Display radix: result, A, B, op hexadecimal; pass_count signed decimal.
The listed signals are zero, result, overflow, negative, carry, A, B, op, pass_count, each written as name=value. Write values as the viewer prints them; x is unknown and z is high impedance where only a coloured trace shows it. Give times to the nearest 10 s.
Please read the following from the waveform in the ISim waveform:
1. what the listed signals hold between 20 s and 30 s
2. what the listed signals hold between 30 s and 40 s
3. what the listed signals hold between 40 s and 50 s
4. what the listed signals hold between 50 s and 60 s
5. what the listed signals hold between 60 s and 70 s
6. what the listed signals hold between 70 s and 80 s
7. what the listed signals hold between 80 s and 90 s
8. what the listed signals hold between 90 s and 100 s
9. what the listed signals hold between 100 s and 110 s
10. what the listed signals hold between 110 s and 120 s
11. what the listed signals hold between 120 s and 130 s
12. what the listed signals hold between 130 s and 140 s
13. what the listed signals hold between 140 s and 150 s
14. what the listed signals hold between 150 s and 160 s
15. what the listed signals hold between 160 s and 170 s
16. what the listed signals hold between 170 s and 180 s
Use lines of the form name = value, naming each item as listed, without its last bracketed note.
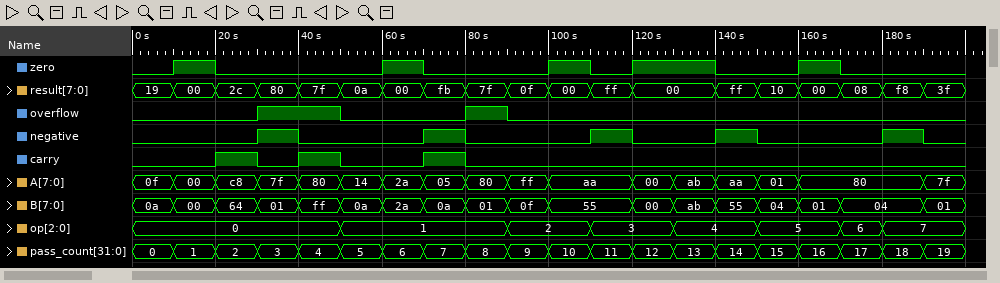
what the listed signals hold between 20 s and 30 s = zero=0, result=2c, overflow=0, negative=0, carry=1, A=c8, B=64, op=0, pass_count=2
what the listed signals hold between 30 s and 40 s = zero=0, result=80, overflow=1, negative=1, carry=0, A=7f, B=01, op=0, pass_count=3
what the listed signals hold between 40 s and 50 s = zero=0, result=7f, overflow=1, negative=0, carry=1, A=80, B=ff, op=0, pass_count=4
what the listed signals hold between 50 s and 60 s = zero=0, result=0a, overflow=0, negative=0, carry=0, A=14, B=0a, op=1, pass_count=5
what the listed signals hold between 60 s and 70 s = zero=1, result=00, overflow=0, negative=0, carry=0, A=2a, B=2a, op=1, pass_count=6
what the listed signals hold between 70 s and 80 s = zero=0, result=fb, overflow=0, negative=1, carry=1, A=05, B=0a, op=1, pass_count=7
what the listed signals hold between 80 s and 90 s = zero=0, result=7f, overflow=1, negative=0, carry=0, A=80, B=01, op=1, pass_count=8
what the listed signals hold between 90 s and 100 s = zero=0, result=0f, overflow=0, negative=0, carry=0, A=ff, B=0f, op=2, pass_count=9
what the listed signals hold between 100 s and 110 s = zero=1, result=00, overflow=0, negative=0, carry=0, A=aa, B=55, op=2, pass_count=10
what the listed signals hold between 110 s and 120 s = zero=0, result=ff, overflow=0, negative=1, carry=0, A=aa, B=55, op=3, pass_count=11
what the listed signals hold between 120 s and 130 s = zero=1, result=00, overflow=0, negative=0, carry=0, A=00, B=00, op=3, pass_count=12
what the listed signals hold between 130 s and 140 s = zero=1, result=00, overflow=0, negative=0, carry=0, A=ab, B=ab, op=4, pass_count=13
what the listed signals hold between 140 s and 150 s = zero=0, result=ff, overflow=0, negative=1, carry=0, A=aa, B=55, op=4, pass_count=14
what the listed signals hold between 150 s and 160 s = zero=0, result=10, overflow=0, negative=0, carry=0, A=01, B=04, op=5, pass_count=15
what the listed signals hold between 160 s and 170 s = zero=1, result=00, overflow=0, negative=0, carry=0, A=80, B=01, op=5, pass_count=16
what the listed signals hold between 170 s and 180 s = zero=0, result=08, overflow=0, negative=0, carry=0, A=80, B=04, op=6, pass_count=17
